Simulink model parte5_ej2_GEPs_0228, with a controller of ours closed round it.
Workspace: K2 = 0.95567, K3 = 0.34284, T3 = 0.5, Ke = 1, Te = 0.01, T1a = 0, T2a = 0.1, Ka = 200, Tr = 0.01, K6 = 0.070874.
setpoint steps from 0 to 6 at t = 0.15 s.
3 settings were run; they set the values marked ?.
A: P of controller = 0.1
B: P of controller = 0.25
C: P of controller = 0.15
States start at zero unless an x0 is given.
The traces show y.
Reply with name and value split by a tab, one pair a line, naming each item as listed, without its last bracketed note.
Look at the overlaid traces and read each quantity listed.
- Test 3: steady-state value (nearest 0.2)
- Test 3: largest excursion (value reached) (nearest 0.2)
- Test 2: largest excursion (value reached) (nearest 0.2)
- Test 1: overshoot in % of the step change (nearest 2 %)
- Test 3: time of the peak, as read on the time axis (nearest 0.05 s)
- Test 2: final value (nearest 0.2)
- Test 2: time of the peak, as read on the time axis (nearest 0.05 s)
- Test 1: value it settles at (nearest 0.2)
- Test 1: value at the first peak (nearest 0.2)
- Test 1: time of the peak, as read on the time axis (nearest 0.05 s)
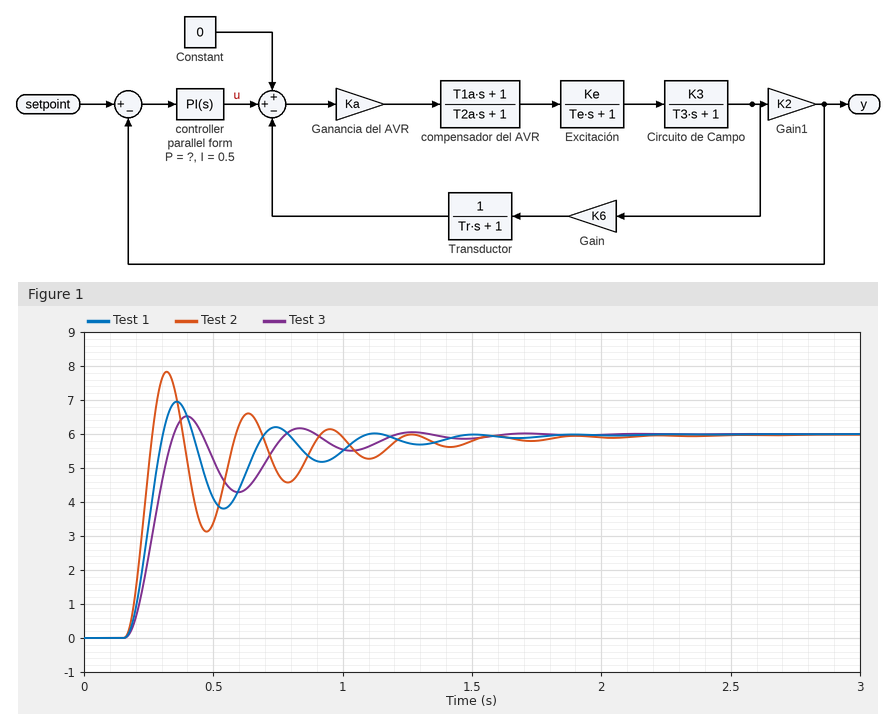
Test 3: steady-state value	6.0
Test 3: largest excursion (value reached)	6.6
Test 2: largest excursion (value reached)	7.8
Test 1: overshoot in % of the step change	16 %
Test 3: time of the peak, as read on the time axis	0.40 s
Test 2: final value	6.0
Test 2: time of the peak, as read on the time axis	0.30 s
Test 1: value it settles at	6.0
Test 1: value at the first peak	7.0
Test 1: time of the peak, as read on the time axis	0.35 s
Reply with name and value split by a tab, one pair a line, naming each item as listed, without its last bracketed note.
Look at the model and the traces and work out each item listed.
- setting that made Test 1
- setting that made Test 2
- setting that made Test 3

setting that made Test 1	C
setting that made Test 2	B
setting that made Test 3	A
